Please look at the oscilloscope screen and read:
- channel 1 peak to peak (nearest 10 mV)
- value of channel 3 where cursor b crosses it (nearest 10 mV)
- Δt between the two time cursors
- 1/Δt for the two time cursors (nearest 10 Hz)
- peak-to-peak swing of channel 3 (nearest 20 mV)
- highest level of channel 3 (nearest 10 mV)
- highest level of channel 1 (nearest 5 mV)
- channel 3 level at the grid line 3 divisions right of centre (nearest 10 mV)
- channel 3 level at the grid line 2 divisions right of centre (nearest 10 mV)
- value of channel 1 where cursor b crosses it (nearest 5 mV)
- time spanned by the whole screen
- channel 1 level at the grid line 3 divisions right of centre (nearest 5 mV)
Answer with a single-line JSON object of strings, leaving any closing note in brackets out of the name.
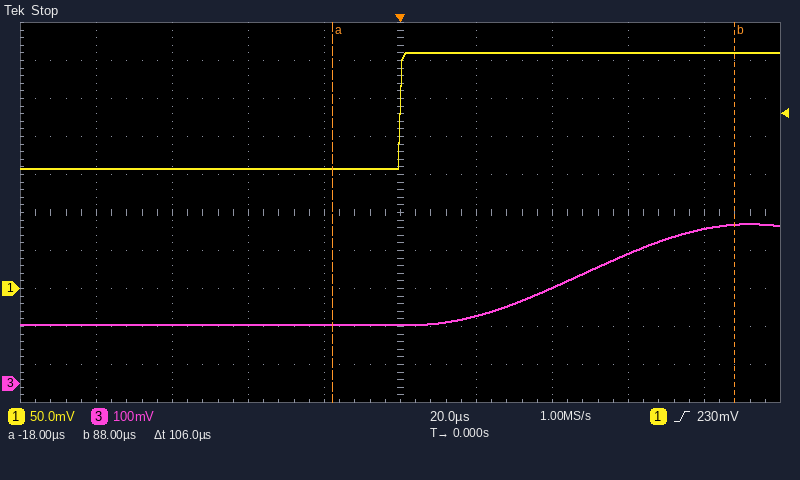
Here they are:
{"channel 1 peak to peak": "150 mV", "value of channel 3 where cursor b crosses it": "420 mV", "Δt between the two time cursors": "106 µs", "1/Δt for the two time cursors": "9.43 kHz", "peak-to-peak swing of channel 3": "260 mV", "highest level of channel 3": "420 mV", "highest level of channel 1": "310 mV", "channel 3 level at the grid line 3 divisions right of centre": "340 mV", "channel 3 level at the grid line 2 divisions right of centre": "250 mV", "value of channel 1 where cursor b crosses it": "310 mV", "time spanned by the whole screen": "200 µs", "channel 1 level at the grid line 3 divisions right of centre": "310 mV"}
